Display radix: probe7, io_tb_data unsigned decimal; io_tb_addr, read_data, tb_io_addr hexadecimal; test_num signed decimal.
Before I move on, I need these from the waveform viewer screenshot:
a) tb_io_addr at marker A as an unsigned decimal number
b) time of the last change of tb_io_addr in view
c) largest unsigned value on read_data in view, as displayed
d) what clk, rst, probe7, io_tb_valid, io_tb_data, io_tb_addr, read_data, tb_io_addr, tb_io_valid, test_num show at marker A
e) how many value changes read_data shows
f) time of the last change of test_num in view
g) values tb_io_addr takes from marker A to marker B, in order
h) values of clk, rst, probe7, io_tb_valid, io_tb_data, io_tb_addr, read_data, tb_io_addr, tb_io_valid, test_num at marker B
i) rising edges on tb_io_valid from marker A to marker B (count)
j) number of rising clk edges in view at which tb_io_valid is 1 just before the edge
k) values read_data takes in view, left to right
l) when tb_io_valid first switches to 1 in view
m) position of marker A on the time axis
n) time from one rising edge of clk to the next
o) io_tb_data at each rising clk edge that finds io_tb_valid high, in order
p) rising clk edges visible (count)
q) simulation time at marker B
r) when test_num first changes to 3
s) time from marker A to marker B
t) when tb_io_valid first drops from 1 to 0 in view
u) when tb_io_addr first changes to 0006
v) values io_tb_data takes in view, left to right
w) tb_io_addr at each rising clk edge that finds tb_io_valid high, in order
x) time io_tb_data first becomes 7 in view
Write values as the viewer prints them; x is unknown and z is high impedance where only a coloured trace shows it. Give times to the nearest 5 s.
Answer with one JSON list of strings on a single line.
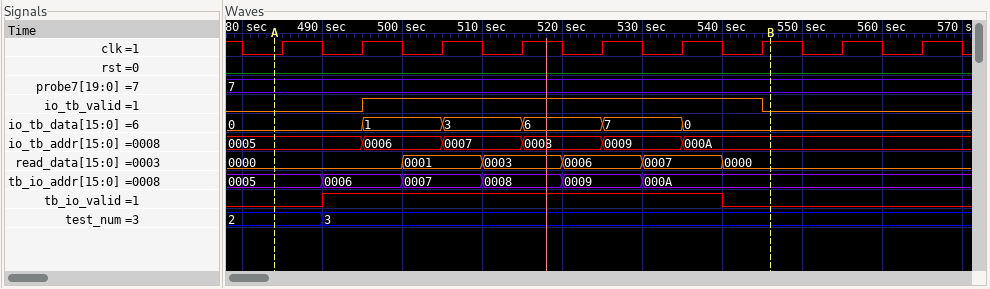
["5", "530 s", "0007", "clk=0, rst=0, probe7=7, io_tb_valid=0, io_tb_data=0, io_tb_addr=0005, read_data=0000, tb_io_addr=0005, tb_io_valid=0, test_num=2", "5", "490 s", "0005, 0006, 0007, 0008, 0009, 000A", "clk=1, rst=0, probe7=7, io_tb_valid=0, io_tb_data=0, io_tb_addr=000A, read_data=0000, tb_io_addr=000A, tb_io_valid=0, test_num=3", "1", "5", "0000, 0001, 0003, 0006, 0007, 0000", "490 s", "485 s", "10 s", "1, 3, 6, 7, 0", "9", "545 s", "490 s", "60 s", "540 s", "490 s", "0, 1, 3, 6, 7, 0", "0006, 0007, 0008, 0009, 000A", "525 s"]
